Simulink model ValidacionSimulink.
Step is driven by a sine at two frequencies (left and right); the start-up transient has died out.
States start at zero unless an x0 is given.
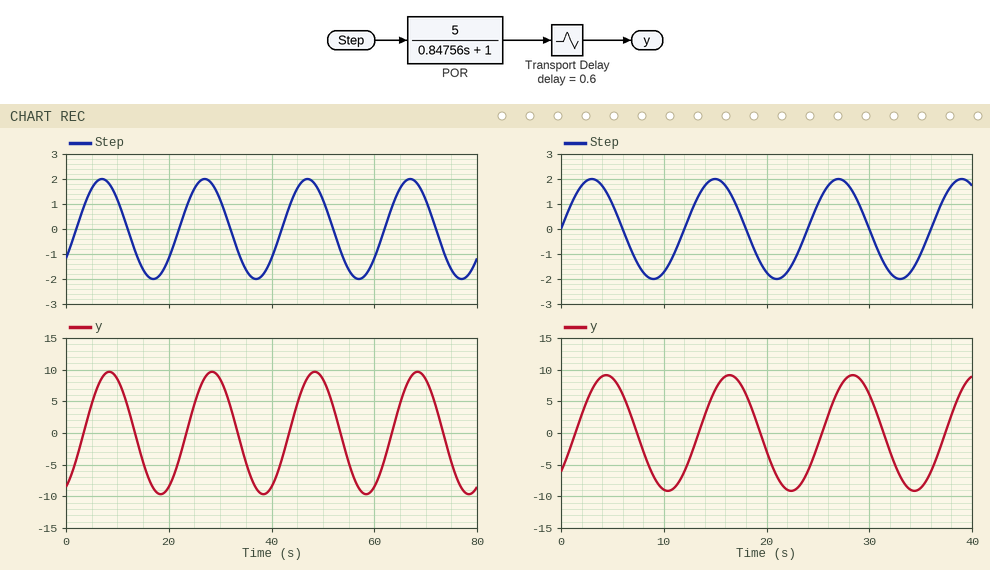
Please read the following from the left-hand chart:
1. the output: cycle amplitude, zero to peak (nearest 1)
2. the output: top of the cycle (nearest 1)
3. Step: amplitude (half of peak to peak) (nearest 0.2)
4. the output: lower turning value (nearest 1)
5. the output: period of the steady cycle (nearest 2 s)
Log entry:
10
10
2.0
-10
20 s
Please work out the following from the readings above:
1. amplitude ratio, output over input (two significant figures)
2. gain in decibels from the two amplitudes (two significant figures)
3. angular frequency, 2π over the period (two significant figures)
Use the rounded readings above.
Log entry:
5.0
14 dB
0.31 rad/s
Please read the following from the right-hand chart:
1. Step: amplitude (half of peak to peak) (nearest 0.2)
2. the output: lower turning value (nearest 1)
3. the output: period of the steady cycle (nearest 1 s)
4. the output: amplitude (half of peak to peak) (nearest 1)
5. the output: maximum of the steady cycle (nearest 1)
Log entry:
2.0
-9
12 s
9
9
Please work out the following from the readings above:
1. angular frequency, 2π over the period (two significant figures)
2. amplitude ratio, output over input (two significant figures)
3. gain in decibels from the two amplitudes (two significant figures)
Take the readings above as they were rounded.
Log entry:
0.52 rad/s
4.5
13 dB
